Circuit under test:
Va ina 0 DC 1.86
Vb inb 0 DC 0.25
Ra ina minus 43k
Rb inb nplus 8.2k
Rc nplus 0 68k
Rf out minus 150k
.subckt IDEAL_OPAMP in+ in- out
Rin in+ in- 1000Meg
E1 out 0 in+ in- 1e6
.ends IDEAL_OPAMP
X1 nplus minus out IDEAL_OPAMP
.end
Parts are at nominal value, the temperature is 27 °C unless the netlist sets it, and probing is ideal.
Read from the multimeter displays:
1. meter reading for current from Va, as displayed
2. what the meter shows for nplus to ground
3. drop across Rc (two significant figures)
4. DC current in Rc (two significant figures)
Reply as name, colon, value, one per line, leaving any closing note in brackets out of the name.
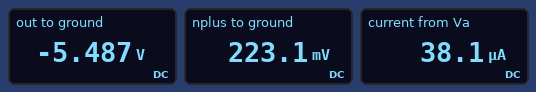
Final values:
meter reading for current from Va, as displayed: 38.1 µA
what the meter shows for nplus to ground: 223.1 mV
drop across Rc: 220 mV
DC current in Rc: 3.3 µA
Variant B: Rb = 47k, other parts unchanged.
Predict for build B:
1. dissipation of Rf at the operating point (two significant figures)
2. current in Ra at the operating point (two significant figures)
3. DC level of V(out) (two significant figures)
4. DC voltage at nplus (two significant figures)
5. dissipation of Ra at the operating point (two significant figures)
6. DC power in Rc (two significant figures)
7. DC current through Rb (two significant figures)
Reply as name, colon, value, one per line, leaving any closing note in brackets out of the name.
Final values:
dissipation of Rf at the operating point: 240 µW
current in Ra at the operating point: 40 µA
DC level of V(out): -5.8 V
DC voltage at nplus: 150 mV
dissipation of Ra at the operating point: 68 µW
DC power in Rc: 320 nW
DC current through Rb: 2.2 µA
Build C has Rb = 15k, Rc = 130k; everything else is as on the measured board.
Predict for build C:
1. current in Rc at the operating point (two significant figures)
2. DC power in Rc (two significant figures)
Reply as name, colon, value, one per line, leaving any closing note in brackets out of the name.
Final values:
current in Rc at the operating point: 1.7 µA
DC power in Rc: 390 nW
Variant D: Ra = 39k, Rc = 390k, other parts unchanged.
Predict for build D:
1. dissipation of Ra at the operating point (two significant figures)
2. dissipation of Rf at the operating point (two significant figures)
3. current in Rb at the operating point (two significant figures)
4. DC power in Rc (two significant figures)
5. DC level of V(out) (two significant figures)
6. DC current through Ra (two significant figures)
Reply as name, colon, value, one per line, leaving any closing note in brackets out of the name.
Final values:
dissipation of Ra at the operating point: 67 µW
dissipation of Rf at the operating point: 260 µW
current in Rb at the operating point: 630 nA
DC power in Rc: 150 nW
DC level of V(out): -6.0 V
DC current through Ra: 41 µA
